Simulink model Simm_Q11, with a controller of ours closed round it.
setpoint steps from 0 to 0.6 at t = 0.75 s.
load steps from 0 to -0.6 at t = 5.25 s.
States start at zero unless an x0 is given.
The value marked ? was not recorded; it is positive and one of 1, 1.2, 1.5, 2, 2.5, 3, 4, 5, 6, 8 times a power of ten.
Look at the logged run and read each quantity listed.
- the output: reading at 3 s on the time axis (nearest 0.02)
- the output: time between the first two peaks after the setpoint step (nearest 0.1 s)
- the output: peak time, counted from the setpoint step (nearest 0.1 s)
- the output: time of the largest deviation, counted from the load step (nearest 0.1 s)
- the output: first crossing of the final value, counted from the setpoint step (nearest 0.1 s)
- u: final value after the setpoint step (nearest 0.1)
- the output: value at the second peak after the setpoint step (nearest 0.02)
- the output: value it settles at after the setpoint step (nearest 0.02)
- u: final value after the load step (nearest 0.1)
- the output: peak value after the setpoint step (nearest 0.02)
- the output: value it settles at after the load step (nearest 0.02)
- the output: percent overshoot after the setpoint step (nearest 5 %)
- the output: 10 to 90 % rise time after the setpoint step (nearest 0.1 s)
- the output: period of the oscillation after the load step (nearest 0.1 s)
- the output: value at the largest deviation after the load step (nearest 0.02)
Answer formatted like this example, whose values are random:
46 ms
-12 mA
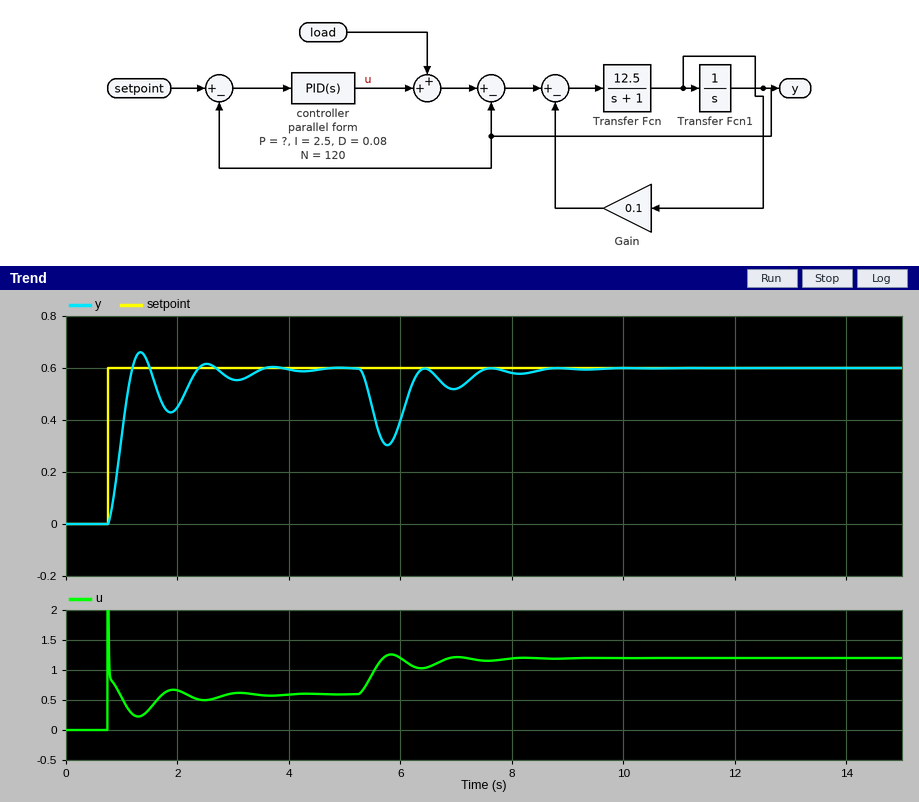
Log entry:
0.56
1.2 s
0.6 s
0.5 s
0.4 s
0.6
0.62
0.60
1.2
0.66
0.60
10 %
0.3 s
1.2 s
0.30
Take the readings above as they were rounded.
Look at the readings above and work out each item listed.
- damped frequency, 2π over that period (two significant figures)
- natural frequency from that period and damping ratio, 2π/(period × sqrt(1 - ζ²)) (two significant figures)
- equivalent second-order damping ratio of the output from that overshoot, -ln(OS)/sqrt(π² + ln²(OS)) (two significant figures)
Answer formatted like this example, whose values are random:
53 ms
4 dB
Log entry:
5.2 rad/s
6.5 rad/s
0.59
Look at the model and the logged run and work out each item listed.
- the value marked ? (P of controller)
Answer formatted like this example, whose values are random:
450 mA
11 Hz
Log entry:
1.5
